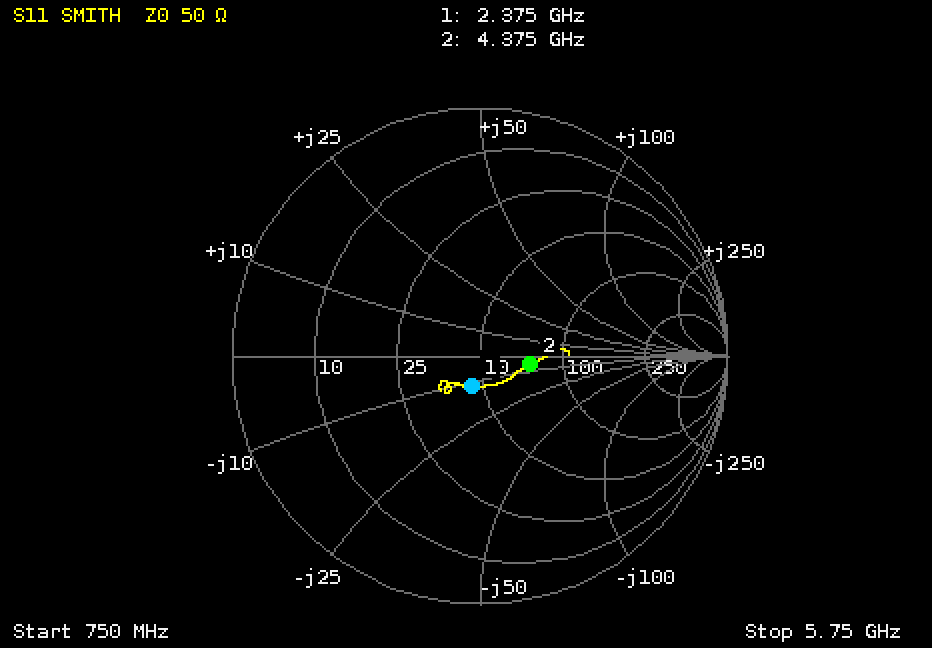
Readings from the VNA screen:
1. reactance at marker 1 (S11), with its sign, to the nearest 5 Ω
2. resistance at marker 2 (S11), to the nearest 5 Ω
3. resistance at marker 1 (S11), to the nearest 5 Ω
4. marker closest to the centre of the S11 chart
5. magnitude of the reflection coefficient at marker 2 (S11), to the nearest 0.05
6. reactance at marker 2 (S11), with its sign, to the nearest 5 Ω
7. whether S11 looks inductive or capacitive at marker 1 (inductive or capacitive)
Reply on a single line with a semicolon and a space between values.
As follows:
-10 Ω; 75 Ω; 45 Ω; marker 1; 0.20; -5 Ω; capacitive
